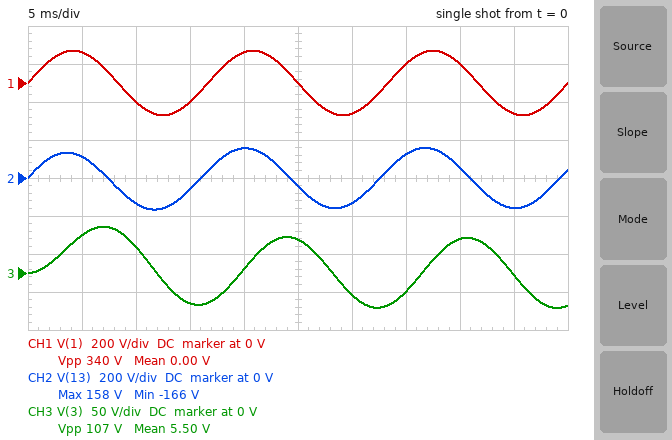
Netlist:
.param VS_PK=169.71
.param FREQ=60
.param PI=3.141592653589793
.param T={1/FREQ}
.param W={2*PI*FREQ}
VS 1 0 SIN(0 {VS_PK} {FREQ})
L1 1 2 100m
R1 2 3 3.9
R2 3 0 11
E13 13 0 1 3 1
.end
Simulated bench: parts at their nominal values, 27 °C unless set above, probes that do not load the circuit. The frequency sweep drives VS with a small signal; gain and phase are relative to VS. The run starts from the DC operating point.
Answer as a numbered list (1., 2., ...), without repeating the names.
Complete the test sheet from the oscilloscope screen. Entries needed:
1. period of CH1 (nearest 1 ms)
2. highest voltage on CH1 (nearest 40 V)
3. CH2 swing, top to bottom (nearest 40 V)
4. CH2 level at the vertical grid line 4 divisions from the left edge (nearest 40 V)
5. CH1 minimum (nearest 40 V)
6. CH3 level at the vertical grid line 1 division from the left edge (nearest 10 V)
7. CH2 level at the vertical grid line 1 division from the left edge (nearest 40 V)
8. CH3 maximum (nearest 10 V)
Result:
1. 17 ms
2. 160 V
3. 320 V
4. 160 V
5. -160 V
6. 50 V
7. 120 V
8. 60 V
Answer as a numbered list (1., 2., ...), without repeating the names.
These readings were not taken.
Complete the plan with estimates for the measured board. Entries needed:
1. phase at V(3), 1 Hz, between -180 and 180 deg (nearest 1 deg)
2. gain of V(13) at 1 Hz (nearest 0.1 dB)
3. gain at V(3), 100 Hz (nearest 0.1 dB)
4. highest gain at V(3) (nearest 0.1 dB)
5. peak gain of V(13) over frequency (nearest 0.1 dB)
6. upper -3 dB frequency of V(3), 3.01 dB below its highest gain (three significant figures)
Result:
1. -2 deg
2. -11.5 dB
3. -15.4 dB
4. -2.6 dB
5. 0 dB
6. 23.7 Hz
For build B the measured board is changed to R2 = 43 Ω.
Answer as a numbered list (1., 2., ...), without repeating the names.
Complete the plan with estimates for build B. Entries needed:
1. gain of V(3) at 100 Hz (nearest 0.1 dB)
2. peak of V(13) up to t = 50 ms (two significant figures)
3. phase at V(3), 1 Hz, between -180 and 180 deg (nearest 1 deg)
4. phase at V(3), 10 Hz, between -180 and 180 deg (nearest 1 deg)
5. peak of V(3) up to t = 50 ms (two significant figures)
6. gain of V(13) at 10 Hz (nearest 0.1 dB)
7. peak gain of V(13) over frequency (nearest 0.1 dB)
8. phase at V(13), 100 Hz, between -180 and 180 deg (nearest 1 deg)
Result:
1. -5.2 dB
2. 110 V
3. -1 deg
4. -8 deg
5. 130 V
6. -16.1 dB
7. 0 dB
8. 33 deg
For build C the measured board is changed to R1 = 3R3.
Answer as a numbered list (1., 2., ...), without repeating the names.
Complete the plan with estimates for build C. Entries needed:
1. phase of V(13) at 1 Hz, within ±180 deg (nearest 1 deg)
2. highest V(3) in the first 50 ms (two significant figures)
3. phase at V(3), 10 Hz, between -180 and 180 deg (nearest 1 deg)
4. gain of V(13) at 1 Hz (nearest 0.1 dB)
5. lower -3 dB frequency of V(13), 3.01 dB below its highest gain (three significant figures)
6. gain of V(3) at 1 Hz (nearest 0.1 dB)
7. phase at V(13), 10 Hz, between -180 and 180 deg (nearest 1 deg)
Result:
1. 8 deg
2. 62 V
3. -24 deg
4. -12.6 dB
5. 21.5 Hz
6. -2.3 dB
7. 39 deg
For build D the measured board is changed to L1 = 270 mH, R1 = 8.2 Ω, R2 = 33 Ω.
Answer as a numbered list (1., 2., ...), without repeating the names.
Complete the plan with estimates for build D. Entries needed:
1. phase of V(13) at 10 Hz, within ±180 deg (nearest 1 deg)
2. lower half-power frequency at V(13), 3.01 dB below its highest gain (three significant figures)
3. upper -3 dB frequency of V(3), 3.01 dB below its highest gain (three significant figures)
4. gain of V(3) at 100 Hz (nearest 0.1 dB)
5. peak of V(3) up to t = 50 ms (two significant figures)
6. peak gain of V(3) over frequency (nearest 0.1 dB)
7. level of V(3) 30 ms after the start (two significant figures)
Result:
1. 42 deg
2. 23.3 Hz
3. 24.3 Hz
4. -14.5 dB
5. 67 V
6. -1.9 dB
7. -32 V
